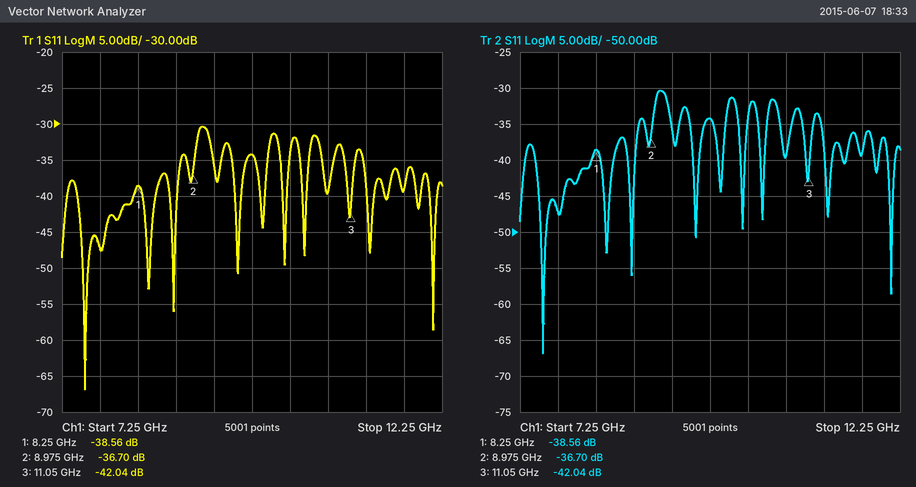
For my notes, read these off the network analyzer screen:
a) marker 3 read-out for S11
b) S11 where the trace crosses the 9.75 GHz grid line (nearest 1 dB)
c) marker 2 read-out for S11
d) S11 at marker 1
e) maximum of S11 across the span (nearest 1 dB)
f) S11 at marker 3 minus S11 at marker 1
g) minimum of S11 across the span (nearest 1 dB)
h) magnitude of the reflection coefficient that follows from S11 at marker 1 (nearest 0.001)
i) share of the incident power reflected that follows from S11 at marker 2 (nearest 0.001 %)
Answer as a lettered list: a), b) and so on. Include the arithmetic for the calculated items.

a) -42.04 dB
b) -34 dB
c) -36.70 dB
d) -38.56 dB
e) -30 dB
f) -42.04 − (-38.56) = -3.48 dB
g) -67 dB
h) 10^(-38.56/20) ≈ 0.012
i) 10^(-36.7/10) ≈ 0.021 %
